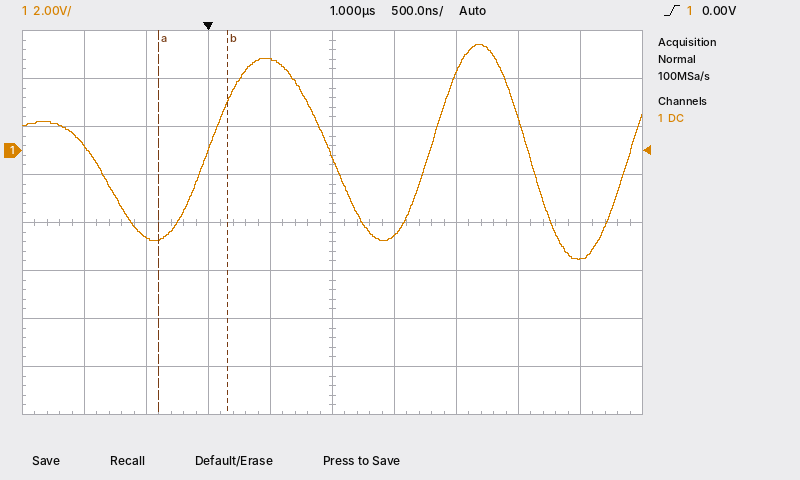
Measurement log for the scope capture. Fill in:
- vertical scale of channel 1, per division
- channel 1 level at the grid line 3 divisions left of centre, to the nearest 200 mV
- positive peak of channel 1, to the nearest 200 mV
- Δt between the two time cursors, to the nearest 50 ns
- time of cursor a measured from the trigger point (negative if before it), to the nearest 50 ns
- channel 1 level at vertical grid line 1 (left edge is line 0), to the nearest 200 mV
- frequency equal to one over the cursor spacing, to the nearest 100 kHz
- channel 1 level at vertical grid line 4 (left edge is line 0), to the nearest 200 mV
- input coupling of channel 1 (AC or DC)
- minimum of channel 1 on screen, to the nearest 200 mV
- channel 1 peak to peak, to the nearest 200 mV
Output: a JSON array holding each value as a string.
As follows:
["2 V", "-3.6 V", "4.4 V", "550 ns", "-400 ns", "200 mV", "1.8 MHz", "3.8 V", "DC", "-4.6 V", "9.0 V"]
